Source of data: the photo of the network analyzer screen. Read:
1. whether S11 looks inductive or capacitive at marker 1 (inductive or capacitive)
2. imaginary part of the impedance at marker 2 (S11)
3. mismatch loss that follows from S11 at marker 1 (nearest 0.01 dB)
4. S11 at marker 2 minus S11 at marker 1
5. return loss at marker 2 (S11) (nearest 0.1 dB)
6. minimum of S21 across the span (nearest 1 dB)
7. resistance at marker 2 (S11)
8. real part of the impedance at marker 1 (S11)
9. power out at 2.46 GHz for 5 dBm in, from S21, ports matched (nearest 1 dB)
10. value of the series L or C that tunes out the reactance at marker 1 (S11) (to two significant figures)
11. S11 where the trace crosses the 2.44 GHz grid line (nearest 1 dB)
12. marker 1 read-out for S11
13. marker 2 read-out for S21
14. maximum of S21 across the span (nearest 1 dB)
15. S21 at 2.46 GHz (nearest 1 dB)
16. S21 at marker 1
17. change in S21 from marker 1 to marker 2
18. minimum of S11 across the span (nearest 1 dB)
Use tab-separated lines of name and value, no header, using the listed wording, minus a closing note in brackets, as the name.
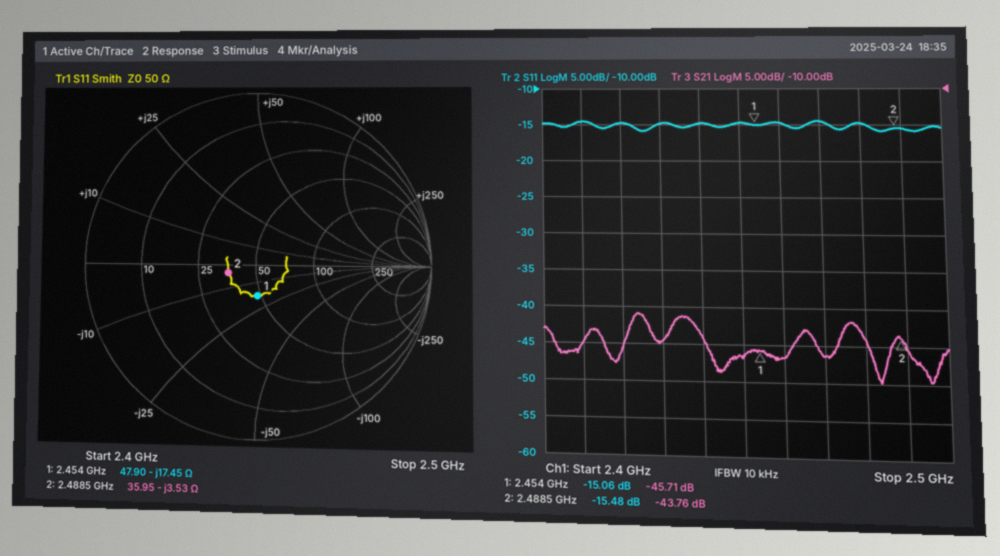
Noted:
whether S11 looks inductive or capacitive at marker 1	capacitive
imaginary part of the impedance at marker 2	-3.53 Ω
mismatch loss that follows from S11 at marker 1	0.14 dB
S11 at marker 2 minus S11 at marker 1	-0.42 dB
return loss at marker 2 (S11)	15.5 dB
minimum of S21 across the span	-50 dB
resistance at marker 2	35.95 Ω
real part of the impedance at marker 1	47.90 Ω
power out at 2.46 GHz for 5 dBm in, from S21, ports matched	-42 dBm
value of the series L or C that tunes out the reactance at marker 1 (S11)	1.1 nH
S11 where the trace crosses the 2.44 GHz grid line	-15 dB
marker 1 read-out for S11	-15.06 dB
marker 2 read-out for S21	-43.76 dB
maximum of S21 across the span	-41 dB
S21 at 2.46 GHz	-47 dB
S21 at marker 1	-45.71 dB
change in S21 from marker 1 to marker 2	1.95 dB
minimum of S11 across the span	-16 dB
